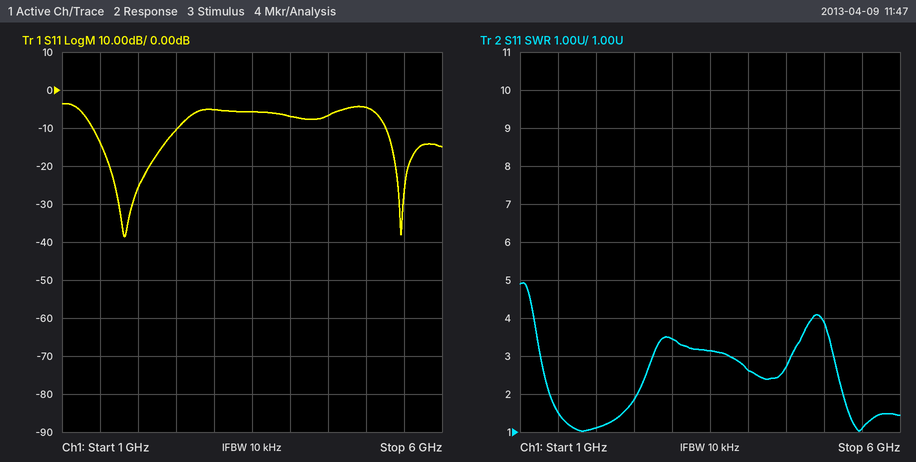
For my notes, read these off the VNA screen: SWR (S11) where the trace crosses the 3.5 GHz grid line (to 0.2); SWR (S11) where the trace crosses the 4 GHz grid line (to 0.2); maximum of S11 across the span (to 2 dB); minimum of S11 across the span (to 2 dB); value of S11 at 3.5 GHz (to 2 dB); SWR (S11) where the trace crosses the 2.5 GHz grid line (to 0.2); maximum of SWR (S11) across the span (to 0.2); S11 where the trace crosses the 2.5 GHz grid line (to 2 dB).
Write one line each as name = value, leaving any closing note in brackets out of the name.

SWR (S11) where the trace crosses the 3.5 GHz grid line = 3.2
SWR (S11) where the trace crosses the 4 GHz grid line = 2.6
maximum of S11 across the span = -4 dB
minimum of S11 across the span = -38 dB
value of S11 at 3.5 GHz = -6 dB
SWR (S11) where the trace crosses the 2.5 GHz grid line = 1.8
maximum of SWR (S11) across the span = 5.0
S11 where the trace crosses the 2.5 GHz grid line = -10 dB
